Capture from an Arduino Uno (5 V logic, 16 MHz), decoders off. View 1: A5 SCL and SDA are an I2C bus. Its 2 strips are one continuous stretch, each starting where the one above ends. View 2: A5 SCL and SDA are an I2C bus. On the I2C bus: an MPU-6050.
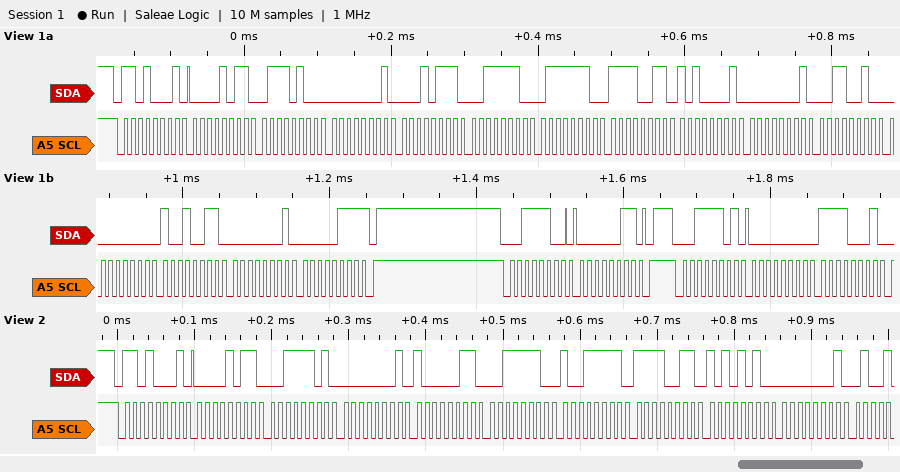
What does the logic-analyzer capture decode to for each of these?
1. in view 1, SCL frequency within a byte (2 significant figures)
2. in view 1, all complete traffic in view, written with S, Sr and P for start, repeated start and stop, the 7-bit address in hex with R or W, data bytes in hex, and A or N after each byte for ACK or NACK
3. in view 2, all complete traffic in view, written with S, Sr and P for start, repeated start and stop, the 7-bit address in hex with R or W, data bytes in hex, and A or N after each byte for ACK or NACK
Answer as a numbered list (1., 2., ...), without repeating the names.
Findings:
1. 100 kHz
2. S 68R A 0B A 74 A 01 A 17 A 3E A 7E A F3 A A1 A 01 A 32 A 00 A 93 A 01 A 07 N P S 1EW A 03 A P S 1ER A 00 A F1 A
3. S 68R A 0B A 3D A 01 A 83 A 3E A 9F A F3 A AA A 01 A
